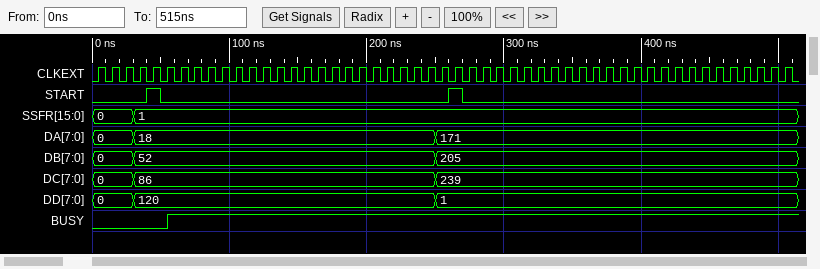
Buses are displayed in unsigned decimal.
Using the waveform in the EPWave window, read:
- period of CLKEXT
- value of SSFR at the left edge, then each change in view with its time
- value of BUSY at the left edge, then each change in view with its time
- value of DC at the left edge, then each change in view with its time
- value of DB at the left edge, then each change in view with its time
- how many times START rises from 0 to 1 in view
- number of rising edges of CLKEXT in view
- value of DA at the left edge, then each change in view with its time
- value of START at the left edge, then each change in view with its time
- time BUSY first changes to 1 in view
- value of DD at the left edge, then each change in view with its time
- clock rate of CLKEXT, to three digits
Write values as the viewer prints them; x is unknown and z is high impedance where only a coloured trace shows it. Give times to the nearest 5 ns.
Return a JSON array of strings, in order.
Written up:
["10 ns", "0, 1 at 30 ns", "0, 1 at 55 ns", "0, 86 at 30 ns, 239 at 250 ns", "0, 52 at 30 ns, 205 at 250 ns", "2", "51", "0, 18 at 30 ns, 171 at 250 ns", "0, 1 at 40 ns, 0 at 50 ns, 1 at 260 ns, 0 at 270 ns", "55 ns", "0, 120 at 30 ns, 1 at 250 ns", "100 MHz"]
